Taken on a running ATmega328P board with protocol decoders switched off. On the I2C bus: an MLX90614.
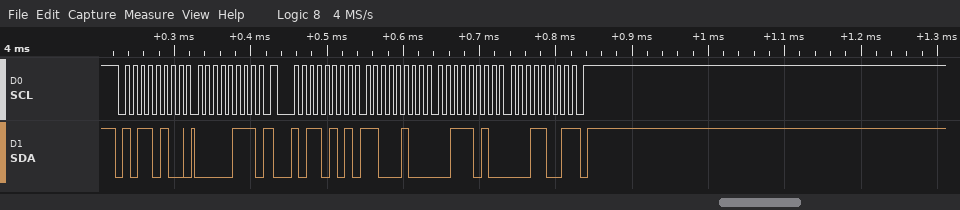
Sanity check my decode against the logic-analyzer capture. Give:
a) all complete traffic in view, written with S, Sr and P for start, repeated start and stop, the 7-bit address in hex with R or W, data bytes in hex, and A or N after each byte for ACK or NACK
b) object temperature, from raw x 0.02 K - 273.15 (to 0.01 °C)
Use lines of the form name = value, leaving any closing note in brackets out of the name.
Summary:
all complete traffic in view, written with S, Sr and P for start, repeated start and stop, the 7-bit address in hex with R or W, data bytes in hex, and A or N after each byte for ACK or NACK = S 5AW A 07 A Sr 5AR A C4 A 3A A 19 N P
object temperature, from raw x 0.02 K - 273.15 = 27.73 °C
